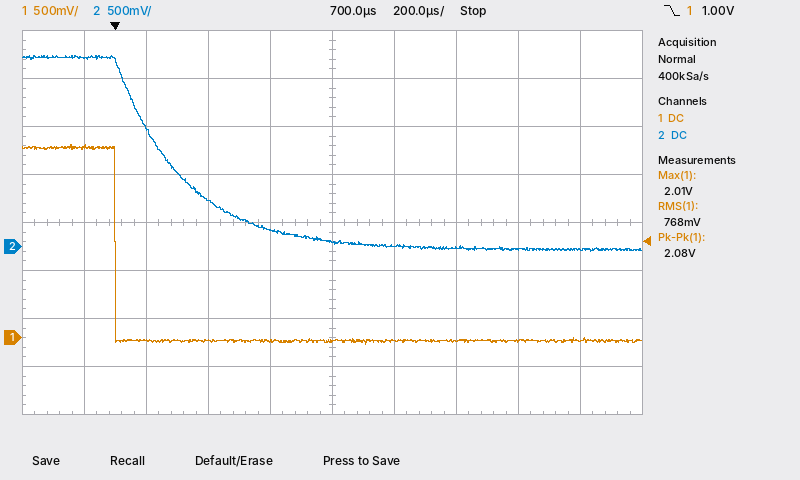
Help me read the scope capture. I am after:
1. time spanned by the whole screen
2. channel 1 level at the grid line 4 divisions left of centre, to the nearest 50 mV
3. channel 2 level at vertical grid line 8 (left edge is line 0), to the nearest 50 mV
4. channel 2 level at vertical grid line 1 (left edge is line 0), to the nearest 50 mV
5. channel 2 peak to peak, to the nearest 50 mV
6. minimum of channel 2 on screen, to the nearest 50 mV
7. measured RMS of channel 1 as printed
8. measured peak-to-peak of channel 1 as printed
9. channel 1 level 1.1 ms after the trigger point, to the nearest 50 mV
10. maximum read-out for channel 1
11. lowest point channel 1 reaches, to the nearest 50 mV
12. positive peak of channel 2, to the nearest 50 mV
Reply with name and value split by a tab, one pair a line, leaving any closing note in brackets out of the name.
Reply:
time spanned by the whole screen	2 ms
channel 1 level at the grid line 4 divisions left of centre, to the nearest 50 mV	2.00 V
channel 2 level at vertical grid line 8 (left edge is line 0), to the nearest 50 mV	-50 mV
channel 2 level at vertical grid line 1 (left edge is line 0), to the nearest 50 mV	1.95 V
channel 2 peak to peak, to the nearest 50 mV	2.05 V
minimum of channel 2 on screen, to the nearest 50 mV	-50 mV
measured RMS of channel 1 as printed	768 mV
measured peak-to-peak of channel 1 as printed	2.08 V
channel 1 level 1.1 ms after the trigger point, to the nearest 50 mV	-50 mV
maximum read-out for channel 1	2.01 V
lowest point channel 1 reaches, to the nearest 50 mV	-50 mV
positive peak of channel 2, to the nearest 50 mV	2.00 V
